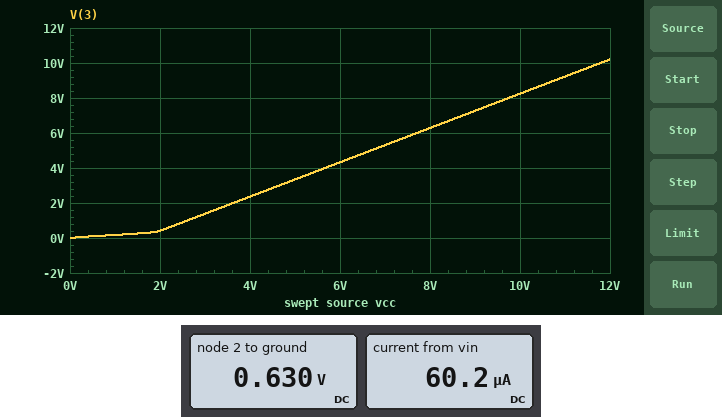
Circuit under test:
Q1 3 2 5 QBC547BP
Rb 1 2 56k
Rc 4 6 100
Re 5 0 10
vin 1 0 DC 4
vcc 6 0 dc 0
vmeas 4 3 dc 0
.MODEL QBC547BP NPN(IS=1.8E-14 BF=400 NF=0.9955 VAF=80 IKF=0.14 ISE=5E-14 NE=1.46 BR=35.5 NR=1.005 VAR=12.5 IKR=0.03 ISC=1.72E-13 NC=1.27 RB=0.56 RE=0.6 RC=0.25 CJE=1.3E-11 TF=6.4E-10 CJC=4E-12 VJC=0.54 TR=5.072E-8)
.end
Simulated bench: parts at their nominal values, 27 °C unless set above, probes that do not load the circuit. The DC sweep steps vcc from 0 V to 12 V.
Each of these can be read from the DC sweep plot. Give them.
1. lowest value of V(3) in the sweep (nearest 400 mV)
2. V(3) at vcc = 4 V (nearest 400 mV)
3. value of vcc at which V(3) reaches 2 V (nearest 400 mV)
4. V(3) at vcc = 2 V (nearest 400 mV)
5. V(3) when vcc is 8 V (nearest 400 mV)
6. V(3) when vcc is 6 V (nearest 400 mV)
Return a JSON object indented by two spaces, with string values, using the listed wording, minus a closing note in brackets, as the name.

{
  "lowest value of V(3) in the sweep": "0 V",
  "V(3) at vcc = 4 V": "2.4 V",
  "value of vcc at which V(3) reaches 2 V": "3.6 V",
  "V(3) at vcc = 2 V": "400 mV",
  "V(3) when vcc is 8 V": "6.4 V",
  "V(3) when vcc is 6 V": "4.4 V"
}
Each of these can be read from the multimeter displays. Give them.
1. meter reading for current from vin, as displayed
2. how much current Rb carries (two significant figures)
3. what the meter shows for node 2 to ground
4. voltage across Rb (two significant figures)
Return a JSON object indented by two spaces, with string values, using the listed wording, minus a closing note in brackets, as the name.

{
  "meter reading for current from vin, as displayed": "60.2 µA",
  "how much current Rb carries": "60 µA",
  "what the meter shows for node 2 to ground": "0.630 V",
  "voltage across Rb": "3.4 V"
}
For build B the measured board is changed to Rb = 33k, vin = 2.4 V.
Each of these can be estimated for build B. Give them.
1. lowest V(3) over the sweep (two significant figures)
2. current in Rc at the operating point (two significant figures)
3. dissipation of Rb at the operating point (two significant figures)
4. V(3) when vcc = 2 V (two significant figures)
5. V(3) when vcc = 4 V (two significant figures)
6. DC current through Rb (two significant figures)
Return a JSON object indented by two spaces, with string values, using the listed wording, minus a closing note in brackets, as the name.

{
  "lowest V(3) over the sweep": "-1.9 mV",
  "current in Rc at the operating point": "19 µA",
  "dissipation of Rb at the operating point": "95 µW",
  "V(3) when vcc = 2 V": "640 mV",
  "V(3) when vcc = 4 V": "2.6 V",
  "DC current through Rb": "54 µA"
}
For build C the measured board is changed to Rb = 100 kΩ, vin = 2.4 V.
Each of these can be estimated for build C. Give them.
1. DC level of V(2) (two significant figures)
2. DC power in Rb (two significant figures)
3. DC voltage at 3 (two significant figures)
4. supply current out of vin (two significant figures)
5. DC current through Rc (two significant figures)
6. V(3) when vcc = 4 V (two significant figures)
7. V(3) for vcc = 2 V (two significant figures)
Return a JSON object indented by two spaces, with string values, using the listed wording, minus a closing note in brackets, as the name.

{
  "DC level of V(2)": "590 mV",
  "DC power in Rb": "33 µW",
  "DC voltage at 3": "-1.0 mV",
  "supply current out of vin": "18 µA",
  "DC current through Rc": "10 µA",
  "V(3) when vcc = 4 V": "3.5 V",
  "V(3) for vcc = 2 V": "1.5 V"
}
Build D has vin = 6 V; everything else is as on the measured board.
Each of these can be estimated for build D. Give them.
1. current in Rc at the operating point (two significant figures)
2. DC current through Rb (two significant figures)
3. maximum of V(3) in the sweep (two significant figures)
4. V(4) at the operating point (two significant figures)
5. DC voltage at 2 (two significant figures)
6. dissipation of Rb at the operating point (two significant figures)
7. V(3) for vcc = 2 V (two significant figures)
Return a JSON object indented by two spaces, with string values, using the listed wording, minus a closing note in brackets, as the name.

{
  "current in Rc at the operating point": "21 µA",
  "DC current through Rb": "96 µA",
  "maximum of V(3) in the sweep": "9.3 V",
  "V(4) at the operating point": "-2.1 mV",
  "DC voltage at 2": "640 mV",
  "dissipation of Rb at the operating point": "510 µW",
  "V(3) for vcc = 2 V": "290 mV"
}
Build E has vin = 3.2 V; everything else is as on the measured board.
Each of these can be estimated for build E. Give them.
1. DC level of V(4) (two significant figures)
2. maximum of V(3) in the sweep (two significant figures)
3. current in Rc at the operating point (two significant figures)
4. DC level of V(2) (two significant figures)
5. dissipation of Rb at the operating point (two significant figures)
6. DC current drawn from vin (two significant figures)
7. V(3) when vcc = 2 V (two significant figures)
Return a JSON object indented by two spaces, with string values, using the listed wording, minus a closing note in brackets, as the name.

{
  "DC level of V(4)": "-1.8 mV",
  "maximum of V(3) in the sweep": "11 V",
  "current in Rc at the operating point": "18 µA",
  "DC level of V(2)": "620 mV",
  "dissipation of Rb at the operating point": "120 µW",
  "DC current drawn from vin": "46 µA",
  "V(3) when vcc = 2 V": "770 mV"
}
